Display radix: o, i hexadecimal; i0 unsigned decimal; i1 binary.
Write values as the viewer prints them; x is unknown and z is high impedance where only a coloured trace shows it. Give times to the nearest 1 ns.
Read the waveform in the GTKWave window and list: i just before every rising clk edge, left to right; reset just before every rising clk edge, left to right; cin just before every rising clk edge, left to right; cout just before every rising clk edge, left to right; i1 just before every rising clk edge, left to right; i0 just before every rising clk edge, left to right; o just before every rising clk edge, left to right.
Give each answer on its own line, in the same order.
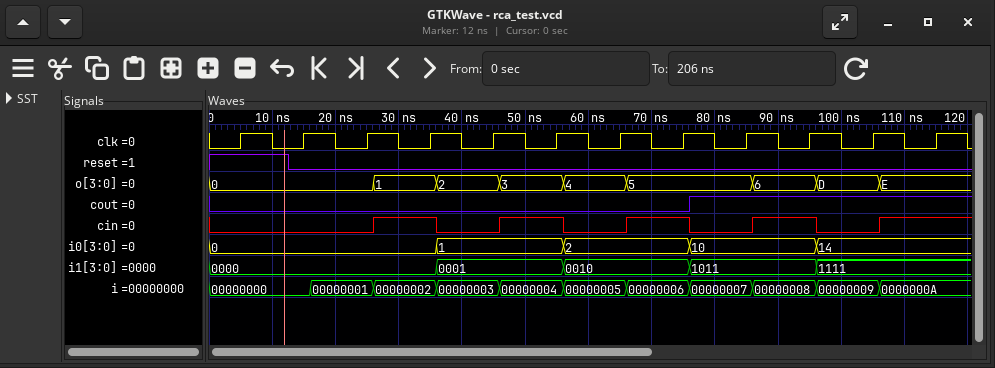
00000000, 00000000, 00000001, 00000002, 00000003, 00000004, 00000005, 00000006, 00000007, 00000008, 00000009, 0000000A
1 0 0 0 0 0 0 0 0 0 0 0
0 0 0 1 0 1 0 1 0 1 0 1
0 0 0 0 0 0 0 0 1 1 1 1
0000, 0000, 0000, 0000, 0001, 0001, 0010, 0010, 1011, 1011, 1111, 1111
0, 0, 0, 0, 1, 1, 2, 2, 10, 10, 14, 14
0, 0, 0, 1, 2, 3, 4, 5, 5, 6, D, E
